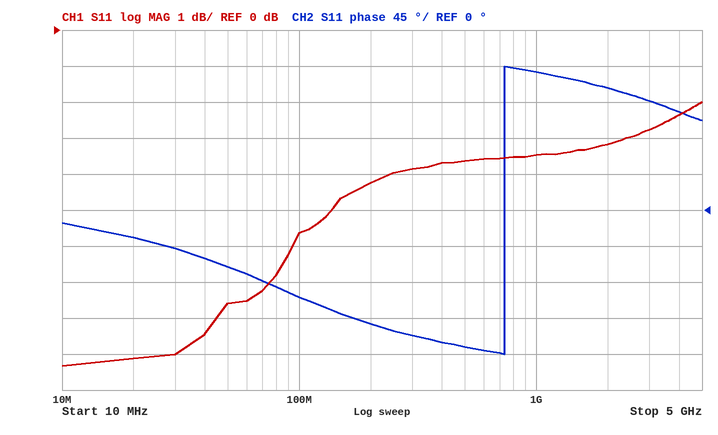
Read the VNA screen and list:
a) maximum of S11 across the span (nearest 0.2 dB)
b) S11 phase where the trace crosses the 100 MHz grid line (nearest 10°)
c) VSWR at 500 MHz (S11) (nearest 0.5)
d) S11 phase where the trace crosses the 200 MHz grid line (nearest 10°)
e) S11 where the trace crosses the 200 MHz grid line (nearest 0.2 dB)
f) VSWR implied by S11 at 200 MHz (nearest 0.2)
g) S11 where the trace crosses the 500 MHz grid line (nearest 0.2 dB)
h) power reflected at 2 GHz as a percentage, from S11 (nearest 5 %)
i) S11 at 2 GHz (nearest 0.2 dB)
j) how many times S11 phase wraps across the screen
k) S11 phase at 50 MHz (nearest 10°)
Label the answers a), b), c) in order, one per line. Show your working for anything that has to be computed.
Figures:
a) -2.0 dB
b) -110°
c) |Γ| = 10^(-3.6/20) = 0.6607; VSWR = (1 + 0.6607)/(1 − 0.6607) ≈ 4.89, so 5.0 to the nearest 0.5
d) -140°
e) -4.2 dB
f) |Γ| = 10^(-4.2/20) = 0.6166; VSWR = (1 + 0.6166)/(1 − 0.6166) ≈ 4.2
g) -3.6 dB
h) 10^(-3.2/10) ≈ 47.9 %, so 50 % to the nearest 5 %
i) -3.2 dB
j) 1
k) -70°
